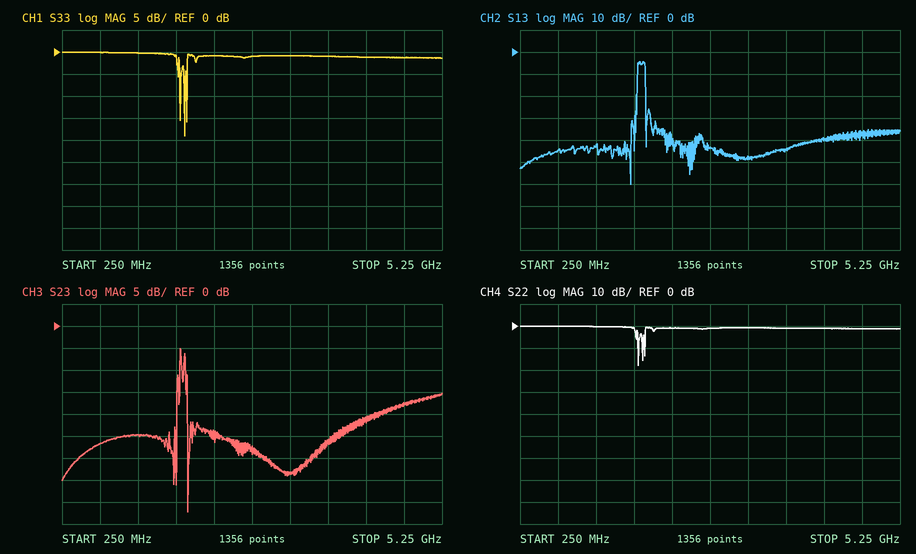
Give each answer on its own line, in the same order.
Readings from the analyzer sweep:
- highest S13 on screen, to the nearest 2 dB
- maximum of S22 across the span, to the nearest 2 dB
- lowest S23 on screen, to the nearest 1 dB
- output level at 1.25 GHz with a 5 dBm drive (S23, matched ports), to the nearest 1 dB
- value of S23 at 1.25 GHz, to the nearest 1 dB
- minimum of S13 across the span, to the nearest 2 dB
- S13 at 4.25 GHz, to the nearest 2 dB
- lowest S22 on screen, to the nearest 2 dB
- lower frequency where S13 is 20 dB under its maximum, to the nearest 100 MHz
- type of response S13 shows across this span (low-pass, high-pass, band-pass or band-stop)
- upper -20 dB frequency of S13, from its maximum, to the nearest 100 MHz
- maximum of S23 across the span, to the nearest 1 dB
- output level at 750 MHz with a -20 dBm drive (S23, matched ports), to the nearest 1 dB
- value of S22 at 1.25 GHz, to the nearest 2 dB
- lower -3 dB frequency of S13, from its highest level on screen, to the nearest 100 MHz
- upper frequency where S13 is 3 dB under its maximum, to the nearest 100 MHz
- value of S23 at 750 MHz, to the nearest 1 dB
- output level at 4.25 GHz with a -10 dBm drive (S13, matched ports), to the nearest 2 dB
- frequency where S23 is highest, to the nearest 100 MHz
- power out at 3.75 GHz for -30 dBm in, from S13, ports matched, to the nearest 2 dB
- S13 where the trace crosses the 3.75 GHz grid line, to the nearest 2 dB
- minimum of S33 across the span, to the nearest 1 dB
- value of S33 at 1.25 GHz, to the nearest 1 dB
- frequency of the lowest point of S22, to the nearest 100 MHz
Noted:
-4 dB
0 dB
-42 dB
-20 dBm
-25 dB
-60 dB
-40 dB
-18 dB
1.8 GHz
band-pass
1.9 GHz
-5 dB
-47 dBm
0 dB
1.8 GHz
1.9 GHz
-27 dB
-50 dBm
1.8 GHz
-74 dBm
-44 dB
-19 dB
0 dB
1.8 GHz
